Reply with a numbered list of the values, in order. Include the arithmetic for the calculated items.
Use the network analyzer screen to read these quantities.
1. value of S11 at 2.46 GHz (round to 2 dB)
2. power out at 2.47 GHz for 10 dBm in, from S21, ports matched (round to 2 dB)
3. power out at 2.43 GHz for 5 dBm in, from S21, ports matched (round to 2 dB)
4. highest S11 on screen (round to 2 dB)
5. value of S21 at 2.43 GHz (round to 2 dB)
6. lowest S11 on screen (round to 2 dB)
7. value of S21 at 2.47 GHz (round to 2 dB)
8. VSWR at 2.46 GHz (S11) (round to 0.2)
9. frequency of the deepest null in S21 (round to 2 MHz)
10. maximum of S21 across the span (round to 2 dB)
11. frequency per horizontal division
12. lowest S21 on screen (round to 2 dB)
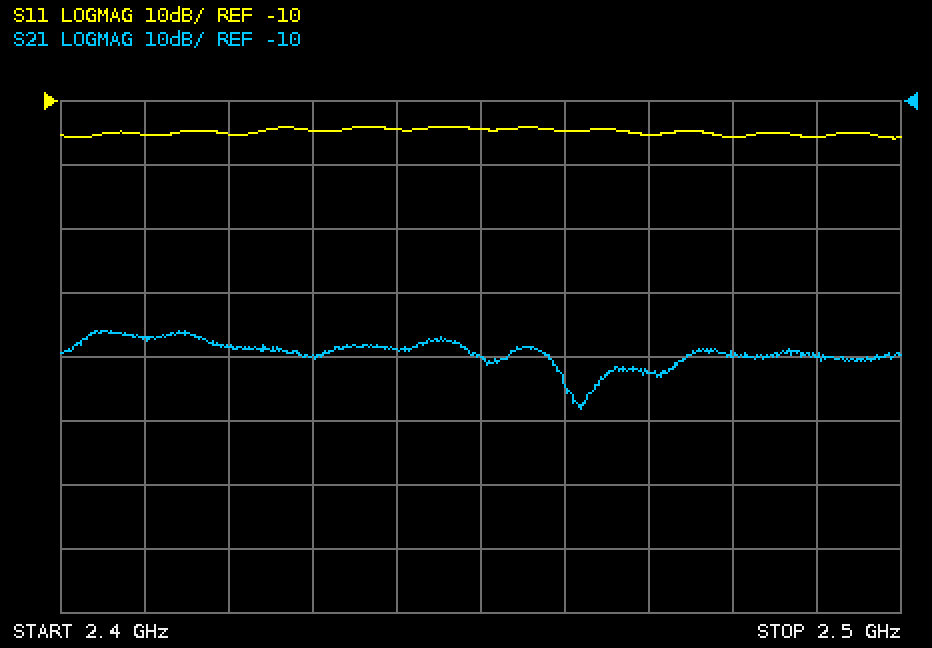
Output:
1. -14 dB
2. 10 dBm + (-52 dB) = -42 dBm
3. 5 dBm + (-50 dB) = -44 dBm
4. -14 dB
5. -50 dB
6. -16 dB
7. -52 dB
8. |Γ| = 10^(-14/20) = 0.1995; VSWR = (1 + 0.1995)/(1 − 0.1995) ≈ 1.50, so 1.4 to the nearest 0.2
9. 2.462 GHz
10. -46 dB
11. 10 MHz
12. -58 dB
